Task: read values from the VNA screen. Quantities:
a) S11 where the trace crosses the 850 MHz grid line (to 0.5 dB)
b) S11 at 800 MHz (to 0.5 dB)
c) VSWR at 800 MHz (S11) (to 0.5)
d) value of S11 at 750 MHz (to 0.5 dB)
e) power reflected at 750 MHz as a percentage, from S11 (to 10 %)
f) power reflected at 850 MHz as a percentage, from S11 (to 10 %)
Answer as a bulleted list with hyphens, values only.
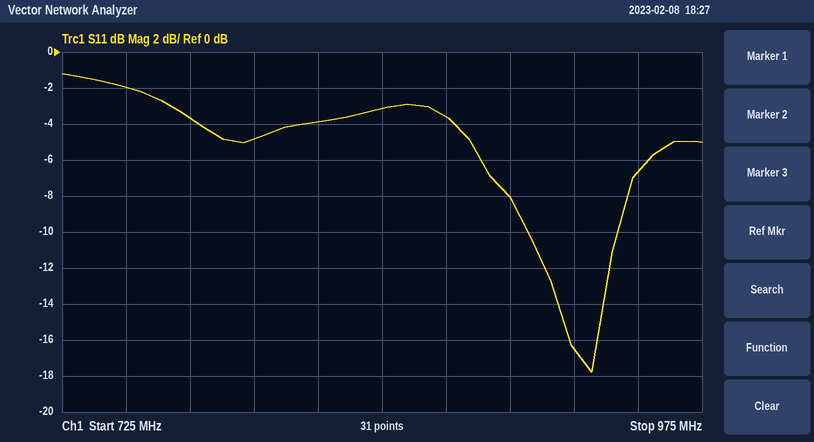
- -3.0 dB
- -5.0 dB
- 3.5
- -2.0 dB
- 60 %
- 50 %
